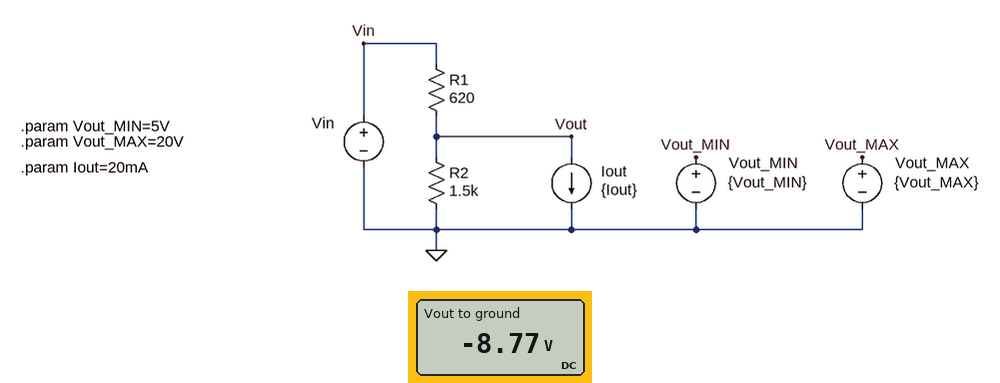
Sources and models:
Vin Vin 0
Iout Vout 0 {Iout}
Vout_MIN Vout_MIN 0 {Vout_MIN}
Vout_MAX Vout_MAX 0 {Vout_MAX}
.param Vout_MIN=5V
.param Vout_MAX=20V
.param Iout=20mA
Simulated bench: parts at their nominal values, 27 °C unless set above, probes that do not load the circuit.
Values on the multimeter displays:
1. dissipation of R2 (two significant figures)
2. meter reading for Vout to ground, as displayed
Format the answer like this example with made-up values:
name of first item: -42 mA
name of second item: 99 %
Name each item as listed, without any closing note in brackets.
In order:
dissipation of R2: 51 mW
meter reading for Vout to ground, as displayed: -8.77 V
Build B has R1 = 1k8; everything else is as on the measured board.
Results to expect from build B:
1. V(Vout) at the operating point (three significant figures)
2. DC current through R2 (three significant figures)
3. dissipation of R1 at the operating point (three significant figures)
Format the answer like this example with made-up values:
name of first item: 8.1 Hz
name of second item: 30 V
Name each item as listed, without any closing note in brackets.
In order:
V(Vout) at the operating point: -16.4 V
DC current through R2: 10.9 mA
dissipation of R1 at the operating point: 149 mW
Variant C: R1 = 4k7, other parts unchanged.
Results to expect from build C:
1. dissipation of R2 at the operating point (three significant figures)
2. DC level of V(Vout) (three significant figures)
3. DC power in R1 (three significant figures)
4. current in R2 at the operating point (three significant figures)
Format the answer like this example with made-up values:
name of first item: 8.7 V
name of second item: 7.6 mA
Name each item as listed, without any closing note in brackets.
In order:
dissipation of R2 at the operating point: 345 mW
DC level of V(Vout): -22.7 V
DC power in R1: 110 mW
current in R2 at the operating point: 15.2 mA
